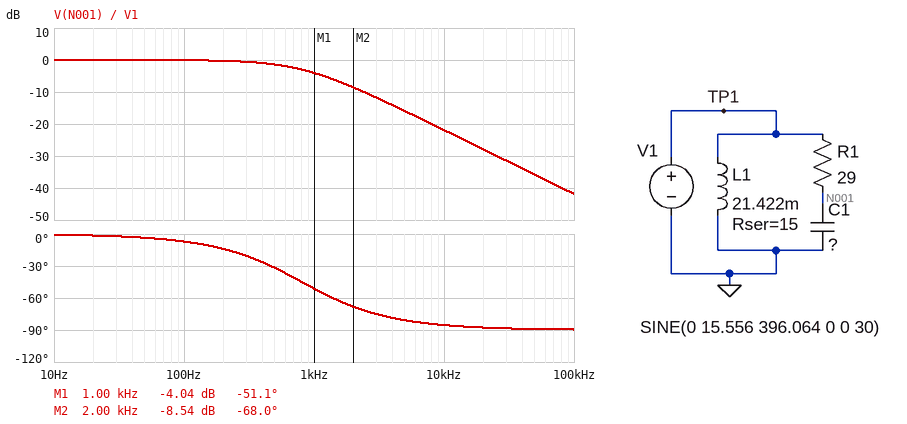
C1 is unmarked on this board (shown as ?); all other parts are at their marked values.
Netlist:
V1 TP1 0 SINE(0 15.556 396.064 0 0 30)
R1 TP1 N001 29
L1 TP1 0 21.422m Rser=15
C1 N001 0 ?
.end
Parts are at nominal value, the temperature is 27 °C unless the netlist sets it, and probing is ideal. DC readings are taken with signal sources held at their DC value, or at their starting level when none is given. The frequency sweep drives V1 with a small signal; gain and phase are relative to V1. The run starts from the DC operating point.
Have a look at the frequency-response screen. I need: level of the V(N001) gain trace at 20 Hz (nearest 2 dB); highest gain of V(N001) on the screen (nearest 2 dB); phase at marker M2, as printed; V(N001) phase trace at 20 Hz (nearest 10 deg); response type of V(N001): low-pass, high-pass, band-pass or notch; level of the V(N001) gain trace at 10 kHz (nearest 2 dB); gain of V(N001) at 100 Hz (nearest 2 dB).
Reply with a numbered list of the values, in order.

1. 0 dB
2. 0 dB
3. -68.0 deg
4. 0 deg
5. low-pass
6. -22 dB
7. 0 dB
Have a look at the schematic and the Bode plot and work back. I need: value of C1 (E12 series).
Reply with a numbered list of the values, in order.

1. 6.8 µF
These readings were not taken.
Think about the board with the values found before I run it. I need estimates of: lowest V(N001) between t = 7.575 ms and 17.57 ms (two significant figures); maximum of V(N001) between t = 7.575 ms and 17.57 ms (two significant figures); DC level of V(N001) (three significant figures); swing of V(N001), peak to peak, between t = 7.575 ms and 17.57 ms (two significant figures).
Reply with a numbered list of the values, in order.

1. -14 V
2. 14 V
3. 7.78 V
4. 28 V
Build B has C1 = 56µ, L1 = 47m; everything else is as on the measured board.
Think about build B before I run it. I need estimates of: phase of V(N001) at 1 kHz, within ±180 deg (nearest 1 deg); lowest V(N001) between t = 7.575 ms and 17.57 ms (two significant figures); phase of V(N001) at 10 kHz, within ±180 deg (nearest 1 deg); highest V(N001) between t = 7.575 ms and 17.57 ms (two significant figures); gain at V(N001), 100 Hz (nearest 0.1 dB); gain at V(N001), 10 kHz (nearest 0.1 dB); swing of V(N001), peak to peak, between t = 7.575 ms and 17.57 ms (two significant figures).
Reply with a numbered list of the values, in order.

1. -84 deg
2. -3.7 V
3. -89 deg
4. 3.8 V
5. -3.1 dB
6. -40.2 dB
7. 7.5 V
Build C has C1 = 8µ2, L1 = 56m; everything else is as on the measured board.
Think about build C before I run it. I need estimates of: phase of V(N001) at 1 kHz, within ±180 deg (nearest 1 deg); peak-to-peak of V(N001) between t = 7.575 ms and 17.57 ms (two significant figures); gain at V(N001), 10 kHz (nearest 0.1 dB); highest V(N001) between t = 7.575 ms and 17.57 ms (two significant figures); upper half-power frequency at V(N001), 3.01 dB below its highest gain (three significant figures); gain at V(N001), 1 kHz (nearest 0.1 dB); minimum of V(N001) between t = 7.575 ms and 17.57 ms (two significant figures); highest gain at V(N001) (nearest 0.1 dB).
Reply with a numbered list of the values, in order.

1. -56 deg
2. 27 V
3. -23.5 dB
4. 13 V
5. 669 Hz
6. -5.1 dB
7. -13 V
8. 0 dB
